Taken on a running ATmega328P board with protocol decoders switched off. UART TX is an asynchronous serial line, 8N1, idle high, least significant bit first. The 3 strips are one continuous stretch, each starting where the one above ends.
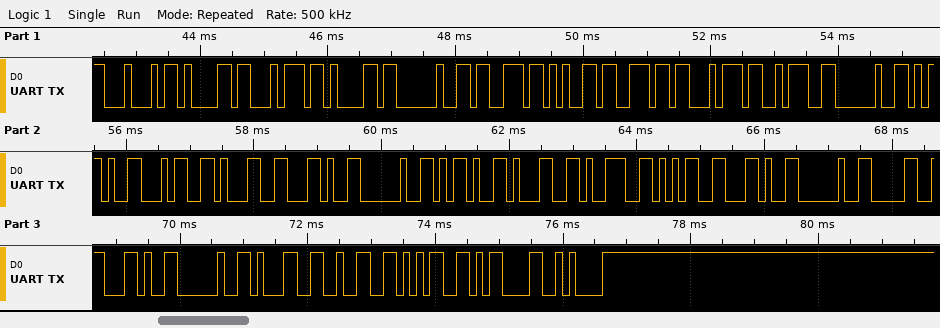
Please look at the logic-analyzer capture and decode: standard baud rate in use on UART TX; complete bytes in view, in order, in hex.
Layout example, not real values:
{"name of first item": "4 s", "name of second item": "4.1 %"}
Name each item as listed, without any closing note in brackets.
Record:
{"standard baud rate in use on UART TX": "9600 baud", "complete bytes in view, in order, in hex": "0x44 0x61 0x74 0x61 0x20 0x73 0x65 0x6E 0x74 0x3A 0x20 0x2D 0x34 0x31 0x2C 0x20 0x2D 0x31 0x39 0x35 0x2C 0x20 0x30 0x2C 0x20 0x31 0x32 0x35 0x0D 0x0A"}
